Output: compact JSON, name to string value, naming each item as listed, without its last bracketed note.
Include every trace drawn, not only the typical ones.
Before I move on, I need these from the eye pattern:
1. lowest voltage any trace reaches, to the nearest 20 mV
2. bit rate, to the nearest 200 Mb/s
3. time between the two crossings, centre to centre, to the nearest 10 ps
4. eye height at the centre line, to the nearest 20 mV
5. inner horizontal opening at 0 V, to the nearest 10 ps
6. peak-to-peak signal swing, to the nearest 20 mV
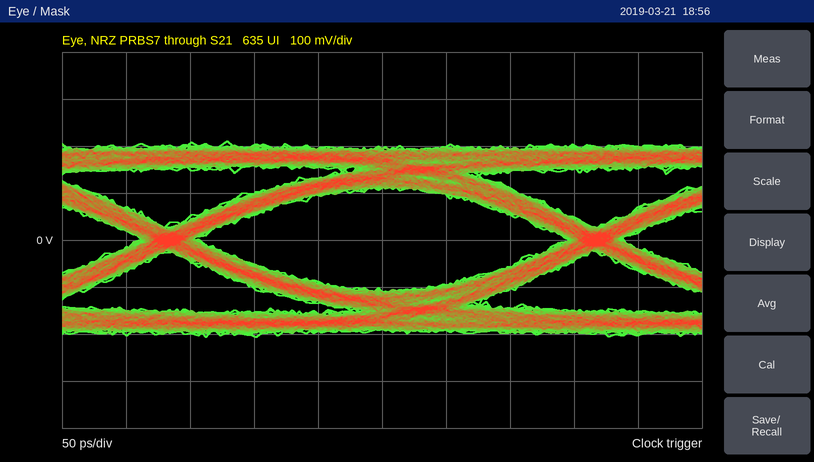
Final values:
{"lowest voltage any trace reaches, to the nearest 20 mV": "-200 mV", "bit rate, to the nearest 200 Mb/s": "3.0 Gb/s", "time between the two crossings, centre to centre, to the nearest 10 ps": "330 ps", "eye height at the centre line, to the nearest 20 mV": "220 mV", "inner horizontal opening at 0 V, to the nearest 10 ps": "290 ps", "peak-to-peak signal swing, to the nearest 20 mV": "420 mV"}
